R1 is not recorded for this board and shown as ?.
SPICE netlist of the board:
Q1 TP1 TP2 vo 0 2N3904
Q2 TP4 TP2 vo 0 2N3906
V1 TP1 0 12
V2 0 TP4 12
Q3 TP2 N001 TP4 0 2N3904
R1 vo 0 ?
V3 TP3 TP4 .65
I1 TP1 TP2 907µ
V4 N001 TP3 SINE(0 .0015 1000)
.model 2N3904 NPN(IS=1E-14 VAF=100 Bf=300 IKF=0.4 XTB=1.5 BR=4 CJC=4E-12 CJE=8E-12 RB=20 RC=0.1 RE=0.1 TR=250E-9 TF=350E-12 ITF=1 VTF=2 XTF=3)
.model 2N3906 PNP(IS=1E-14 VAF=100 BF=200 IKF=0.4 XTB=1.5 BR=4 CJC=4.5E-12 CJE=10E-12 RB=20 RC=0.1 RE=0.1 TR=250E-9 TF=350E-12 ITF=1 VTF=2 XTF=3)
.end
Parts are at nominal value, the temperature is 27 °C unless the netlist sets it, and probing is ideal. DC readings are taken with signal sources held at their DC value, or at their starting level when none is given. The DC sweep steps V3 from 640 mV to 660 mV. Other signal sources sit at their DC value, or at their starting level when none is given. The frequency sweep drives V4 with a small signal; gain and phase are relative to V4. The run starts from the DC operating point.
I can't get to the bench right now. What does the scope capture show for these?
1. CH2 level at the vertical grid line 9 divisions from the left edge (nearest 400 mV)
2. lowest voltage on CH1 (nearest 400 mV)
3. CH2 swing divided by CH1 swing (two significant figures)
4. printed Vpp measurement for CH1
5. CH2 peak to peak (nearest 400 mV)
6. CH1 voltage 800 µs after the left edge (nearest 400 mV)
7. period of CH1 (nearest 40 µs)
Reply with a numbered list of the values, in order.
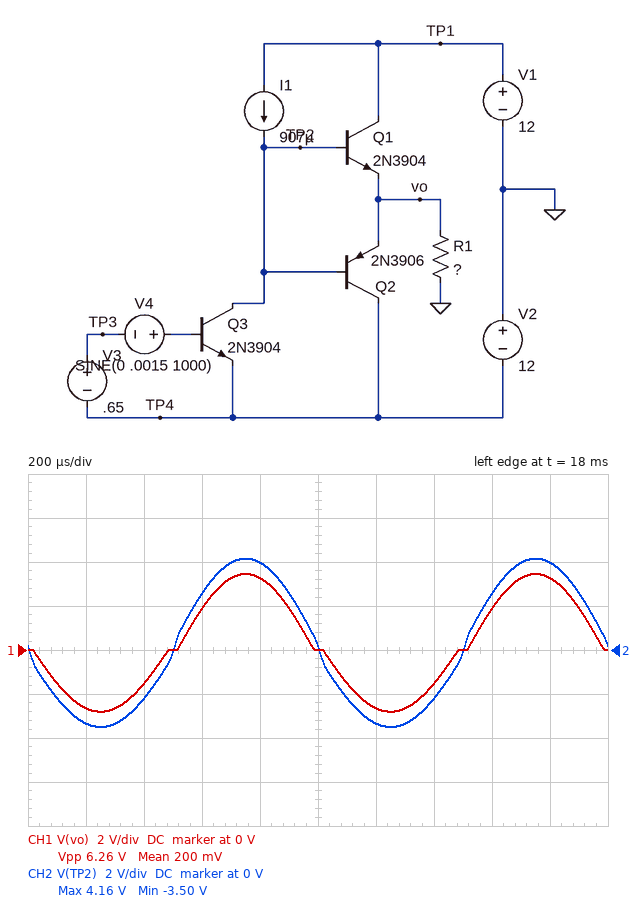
1. 4.0 V
2. -2.8 V
3. 1.2
4. 6.26 V
5. 7.6 V
6. 3.2 V
7. 1.00 ms
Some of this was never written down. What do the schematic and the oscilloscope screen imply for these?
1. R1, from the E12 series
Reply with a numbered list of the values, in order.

1. 560 Ω
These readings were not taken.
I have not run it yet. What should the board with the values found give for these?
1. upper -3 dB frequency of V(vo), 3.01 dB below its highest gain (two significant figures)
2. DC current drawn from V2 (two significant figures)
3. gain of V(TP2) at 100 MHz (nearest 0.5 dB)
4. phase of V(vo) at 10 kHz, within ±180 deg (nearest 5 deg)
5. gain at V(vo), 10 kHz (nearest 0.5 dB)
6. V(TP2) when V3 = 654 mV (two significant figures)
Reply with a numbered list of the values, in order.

1. 59 MHz
2. 910 µA
3. 17.5 dB
4. -100 deg
5. 8.5 dB
6. -8.5 V
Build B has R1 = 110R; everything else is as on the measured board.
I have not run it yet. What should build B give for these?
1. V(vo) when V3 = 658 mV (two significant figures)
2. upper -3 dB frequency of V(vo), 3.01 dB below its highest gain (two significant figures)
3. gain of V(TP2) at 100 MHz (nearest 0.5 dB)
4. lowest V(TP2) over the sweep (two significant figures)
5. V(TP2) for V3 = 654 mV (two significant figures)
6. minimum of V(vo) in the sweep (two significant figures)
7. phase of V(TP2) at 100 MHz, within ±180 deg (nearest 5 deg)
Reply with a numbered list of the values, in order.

1. -5.4 V
2. 200 MHz
3. 11.0 dB
4. -7.5 V
5. -3.4 V
6. -6.7 V
7. 110 deg
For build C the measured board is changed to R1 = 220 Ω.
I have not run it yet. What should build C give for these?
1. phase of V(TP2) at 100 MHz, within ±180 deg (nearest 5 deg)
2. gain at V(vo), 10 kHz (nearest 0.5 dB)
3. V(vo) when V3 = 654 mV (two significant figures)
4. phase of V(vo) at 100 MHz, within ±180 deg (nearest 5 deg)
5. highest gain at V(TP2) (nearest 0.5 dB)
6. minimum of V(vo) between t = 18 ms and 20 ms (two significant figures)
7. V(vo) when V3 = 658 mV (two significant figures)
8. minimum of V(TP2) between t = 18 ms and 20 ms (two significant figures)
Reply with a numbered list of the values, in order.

1. 110 deg
2. 0.5 dB
3. -4.5 V
4. 130 deg
5. 72.5 dB
6. -1.6 V
7. -9.0 V
8. -2.3 V
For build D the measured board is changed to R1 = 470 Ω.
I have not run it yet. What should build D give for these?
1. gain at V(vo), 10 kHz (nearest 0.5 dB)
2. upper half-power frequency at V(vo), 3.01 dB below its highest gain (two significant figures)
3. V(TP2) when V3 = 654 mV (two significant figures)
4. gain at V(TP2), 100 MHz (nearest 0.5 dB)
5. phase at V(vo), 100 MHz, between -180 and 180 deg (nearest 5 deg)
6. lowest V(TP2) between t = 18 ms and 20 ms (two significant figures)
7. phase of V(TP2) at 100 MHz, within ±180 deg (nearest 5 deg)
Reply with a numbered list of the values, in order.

1. 7.0 dB
2. 69 MHz
3. -7.9 V
4. 17.0 dB
5. 110 deg
6. -3.3 V
7. 100 deg
